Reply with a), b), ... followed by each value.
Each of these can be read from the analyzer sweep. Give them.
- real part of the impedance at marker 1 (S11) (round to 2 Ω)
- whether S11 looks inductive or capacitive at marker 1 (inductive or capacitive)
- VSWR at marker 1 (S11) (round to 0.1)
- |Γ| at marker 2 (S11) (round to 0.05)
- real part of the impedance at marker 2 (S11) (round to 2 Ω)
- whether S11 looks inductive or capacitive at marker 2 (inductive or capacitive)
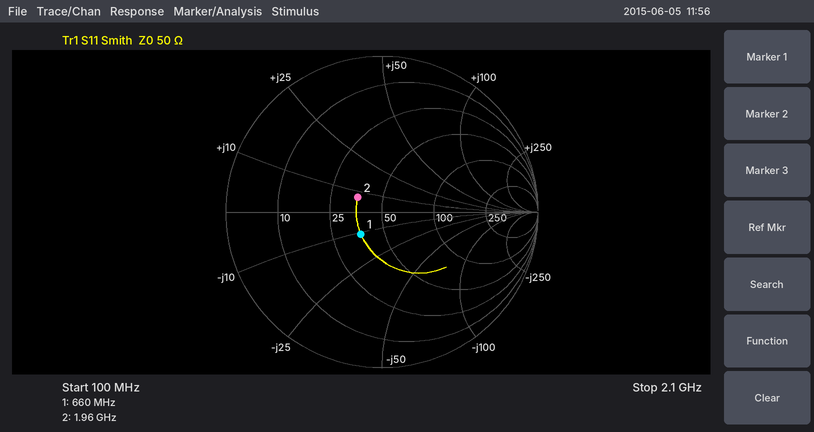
a) 36 Ω
b) capacitive
c) 1.5
d) 0.20
e) 36 Ω
f) inductive
